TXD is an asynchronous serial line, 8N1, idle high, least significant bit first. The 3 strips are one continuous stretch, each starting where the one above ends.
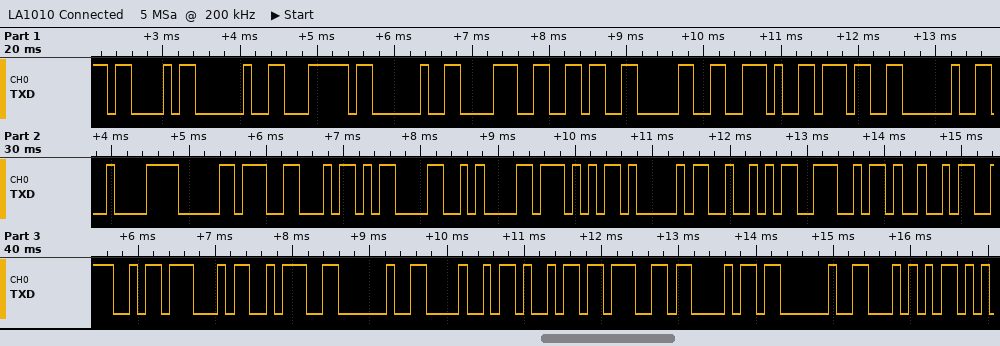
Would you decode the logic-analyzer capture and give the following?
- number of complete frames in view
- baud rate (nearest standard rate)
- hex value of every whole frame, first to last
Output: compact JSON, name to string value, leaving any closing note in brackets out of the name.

{"number of complete frames in view": "30", "baud rate": "9600 baud", "hex value of every whole frame, first to last": "43 20 7C 20 38 36 30 2E 37 20 C2 B0 46 0D 0A 57 41 52 4E 49 4E 47 3A 20 48 69 67 68 20 54"}
